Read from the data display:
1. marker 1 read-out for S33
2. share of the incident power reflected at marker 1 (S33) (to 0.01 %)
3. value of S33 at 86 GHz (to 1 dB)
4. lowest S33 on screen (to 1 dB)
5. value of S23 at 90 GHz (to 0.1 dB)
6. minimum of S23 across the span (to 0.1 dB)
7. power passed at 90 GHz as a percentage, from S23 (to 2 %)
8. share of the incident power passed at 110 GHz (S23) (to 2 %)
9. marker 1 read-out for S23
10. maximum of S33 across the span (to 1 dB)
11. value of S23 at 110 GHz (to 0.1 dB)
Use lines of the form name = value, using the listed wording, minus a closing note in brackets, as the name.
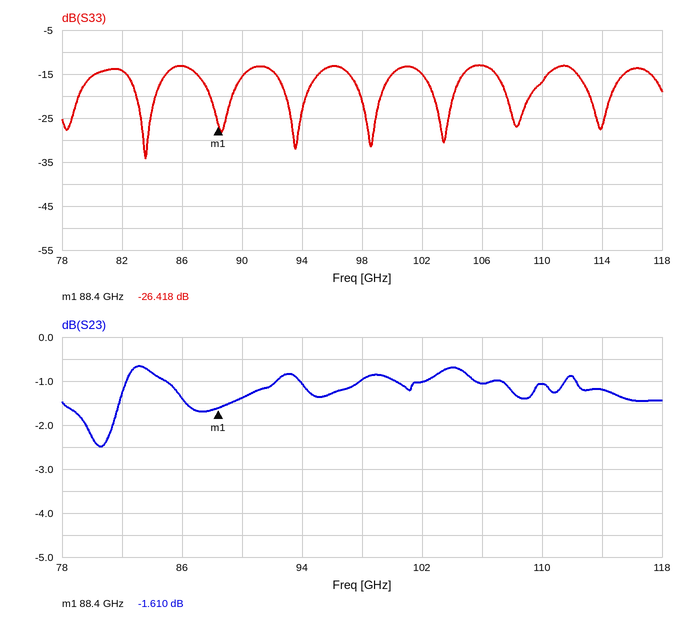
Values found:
marker 1 read-out for S33 = -26.418 dB
share of the incident power reflected at marker 1 (S33) = 0.23 %
value of S33 at 86 GHz = -13 dB
lowest S33 on screen = -34 dB
value of S23 at 90 GHz = -1.4 dB
minimum of S23 across the span = -2.5 dB
power passed at 90 GHz as a percentage, from S23 = 72 %
share of the incident power passed at 110 GHz (S23) = 78 %
marker 1 read-out for S23 = -1.610 dB
maximum of S33 across the span = -13 dB
value of S23 at 110 GHz = -1.1 dB
